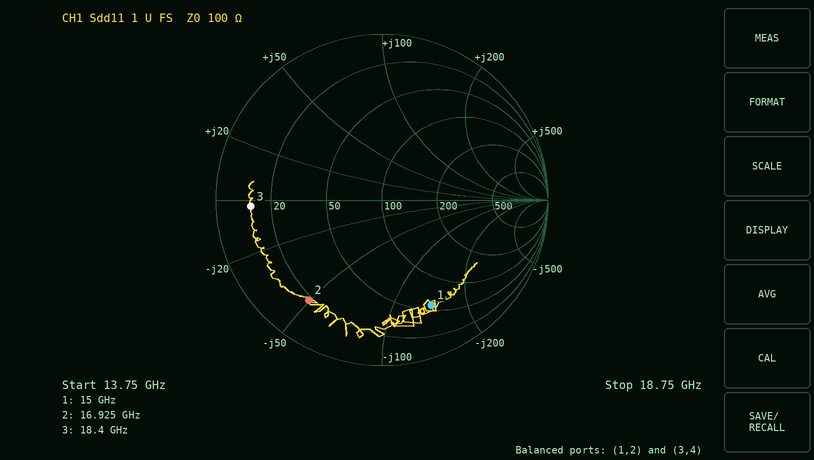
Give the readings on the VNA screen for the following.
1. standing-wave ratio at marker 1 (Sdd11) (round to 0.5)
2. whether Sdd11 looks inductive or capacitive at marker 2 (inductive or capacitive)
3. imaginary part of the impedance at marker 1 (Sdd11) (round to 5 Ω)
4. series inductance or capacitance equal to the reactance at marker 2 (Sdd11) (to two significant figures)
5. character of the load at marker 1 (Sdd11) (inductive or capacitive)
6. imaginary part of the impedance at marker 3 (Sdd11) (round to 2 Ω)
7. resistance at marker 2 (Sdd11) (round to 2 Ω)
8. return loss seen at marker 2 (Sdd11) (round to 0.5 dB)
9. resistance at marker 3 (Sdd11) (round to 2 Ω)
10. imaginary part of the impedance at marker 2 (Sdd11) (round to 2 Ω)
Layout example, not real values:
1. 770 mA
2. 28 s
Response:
1. 5.5
2. capacitive
3. -140 Ω
4. 190 fF
5. capacitive
6. -2 Ω
7. 18 Ω
8. 2.5 dB
9. 12 Ω
10. -50 Ω
